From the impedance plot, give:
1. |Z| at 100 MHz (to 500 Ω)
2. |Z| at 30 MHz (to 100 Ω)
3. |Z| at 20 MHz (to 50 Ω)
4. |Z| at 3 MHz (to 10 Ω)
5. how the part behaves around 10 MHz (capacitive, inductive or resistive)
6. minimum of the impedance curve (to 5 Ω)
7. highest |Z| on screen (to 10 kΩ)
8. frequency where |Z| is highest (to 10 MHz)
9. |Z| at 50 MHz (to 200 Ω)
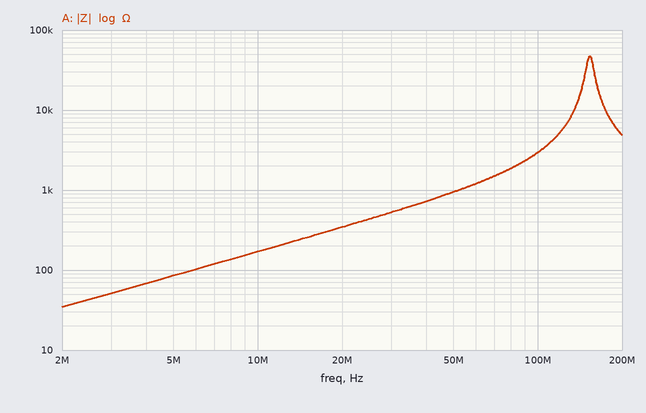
3.0 kΩ
500 Ω
350 Ω
50 Ω
inductive
35 Ω
50 kΩ
150 MHz
1.0 kΩ
